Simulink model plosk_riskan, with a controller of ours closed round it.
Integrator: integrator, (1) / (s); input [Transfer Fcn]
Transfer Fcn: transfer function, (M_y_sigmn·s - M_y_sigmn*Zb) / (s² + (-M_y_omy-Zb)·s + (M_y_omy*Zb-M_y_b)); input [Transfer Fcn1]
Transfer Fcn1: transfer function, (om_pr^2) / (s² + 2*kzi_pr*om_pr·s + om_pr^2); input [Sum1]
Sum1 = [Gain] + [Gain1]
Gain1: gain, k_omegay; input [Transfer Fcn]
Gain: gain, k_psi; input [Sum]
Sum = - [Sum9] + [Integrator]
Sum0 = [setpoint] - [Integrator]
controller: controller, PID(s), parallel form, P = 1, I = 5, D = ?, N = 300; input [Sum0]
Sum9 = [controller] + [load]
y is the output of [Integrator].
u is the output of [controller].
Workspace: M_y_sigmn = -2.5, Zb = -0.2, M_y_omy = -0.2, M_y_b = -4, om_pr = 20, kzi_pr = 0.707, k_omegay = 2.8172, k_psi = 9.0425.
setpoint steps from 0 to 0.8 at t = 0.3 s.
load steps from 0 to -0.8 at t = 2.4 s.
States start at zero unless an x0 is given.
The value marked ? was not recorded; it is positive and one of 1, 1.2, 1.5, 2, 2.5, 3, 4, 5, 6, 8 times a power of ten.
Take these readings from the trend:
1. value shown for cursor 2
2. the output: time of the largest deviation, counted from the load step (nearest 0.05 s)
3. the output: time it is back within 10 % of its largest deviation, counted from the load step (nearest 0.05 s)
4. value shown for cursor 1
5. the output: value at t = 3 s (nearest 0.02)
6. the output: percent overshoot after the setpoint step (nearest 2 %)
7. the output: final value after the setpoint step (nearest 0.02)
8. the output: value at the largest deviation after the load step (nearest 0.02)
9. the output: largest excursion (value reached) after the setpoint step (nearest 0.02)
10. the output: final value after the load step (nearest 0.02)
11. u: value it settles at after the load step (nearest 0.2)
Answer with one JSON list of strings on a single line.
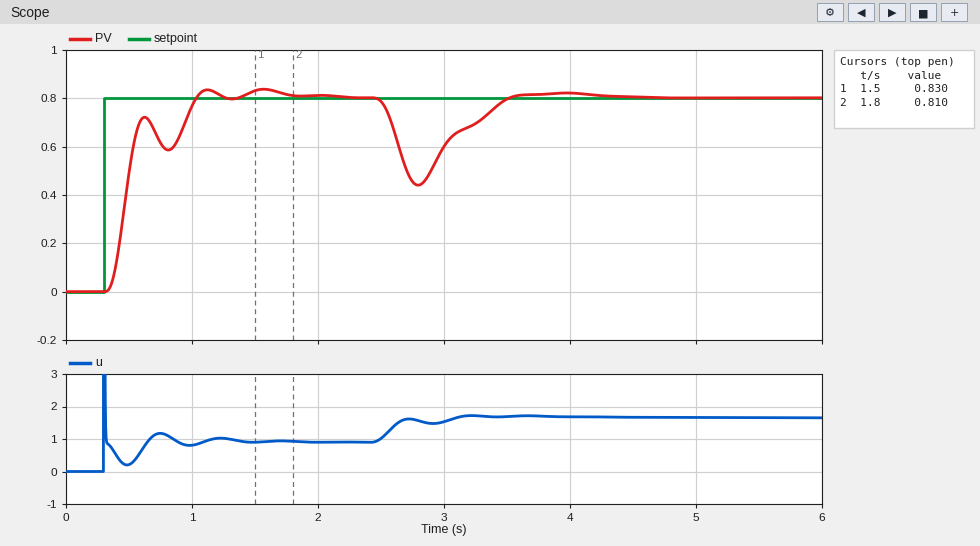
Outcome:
["0.810", "0.40 s", "1.00 s", "0.830", "0.60", "4 %", "0.80", "0.44", "0.84", "0.80", "1.6"]
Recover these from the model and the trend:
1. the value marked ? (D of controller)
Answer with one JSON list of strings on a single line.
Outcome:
["0.2"]
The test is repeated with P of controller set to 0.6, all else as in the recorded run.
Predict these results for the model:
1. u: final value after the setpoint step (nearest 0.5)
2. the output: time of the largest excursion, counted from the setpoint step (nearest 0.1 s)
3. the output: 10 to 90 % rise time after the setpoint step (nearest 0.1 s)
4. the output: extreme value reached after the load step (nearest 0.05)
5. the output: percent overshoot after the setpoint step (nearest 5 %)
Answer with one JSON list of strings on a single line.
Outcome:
["1.0", "1.2 s", "0.6 s", "0.40", "10 %"]
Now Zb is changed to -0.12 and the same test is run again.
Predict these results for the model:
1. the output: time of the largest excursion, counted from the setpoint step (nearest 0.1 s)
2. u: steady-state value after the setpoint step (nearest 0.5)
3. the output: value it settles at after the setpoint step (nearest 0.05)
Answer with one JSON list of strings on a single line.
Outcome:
["1.3 s", "1.0", "0.80"]
